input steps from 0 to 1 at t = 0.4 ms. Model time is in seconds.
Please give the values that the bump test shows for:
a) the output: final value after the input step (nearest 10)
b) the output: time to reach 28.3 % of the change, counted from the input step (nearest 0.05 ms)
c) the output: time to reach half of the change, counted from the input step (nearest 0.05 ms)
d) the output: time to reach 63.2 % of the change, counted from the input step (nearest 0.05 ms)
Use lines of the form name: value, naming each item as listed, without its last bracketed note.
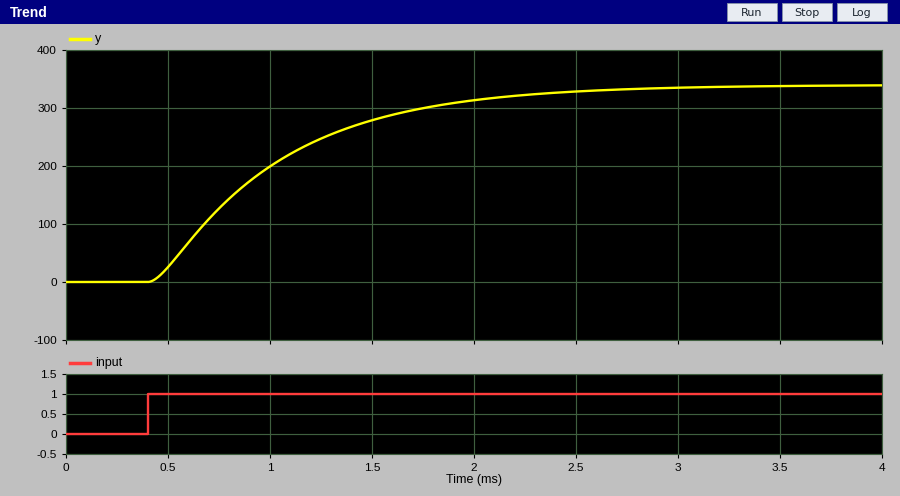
the output: final value after the input step: 340
the output: time to reach 28.3 % of the change, counted from the input step: 0.25 ms
the output: time to reach half of the change, counted from the input step: 0.50 ms
the output: time to reach 63.2 % of the change, counted from the input step: 0.65 ms
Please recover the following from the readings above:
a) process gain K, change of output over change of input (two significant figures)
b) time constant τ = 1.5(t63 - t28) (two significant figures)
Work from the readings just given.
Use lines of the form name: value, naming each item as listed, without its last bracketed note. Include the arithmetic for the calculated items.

process gain K, change of output over change of input: (340 - 0) / 1 = 340
time constant τ = 1.5(t63 - t28): 1.5 × (0.65 - 0.25) = 0.60 ms
